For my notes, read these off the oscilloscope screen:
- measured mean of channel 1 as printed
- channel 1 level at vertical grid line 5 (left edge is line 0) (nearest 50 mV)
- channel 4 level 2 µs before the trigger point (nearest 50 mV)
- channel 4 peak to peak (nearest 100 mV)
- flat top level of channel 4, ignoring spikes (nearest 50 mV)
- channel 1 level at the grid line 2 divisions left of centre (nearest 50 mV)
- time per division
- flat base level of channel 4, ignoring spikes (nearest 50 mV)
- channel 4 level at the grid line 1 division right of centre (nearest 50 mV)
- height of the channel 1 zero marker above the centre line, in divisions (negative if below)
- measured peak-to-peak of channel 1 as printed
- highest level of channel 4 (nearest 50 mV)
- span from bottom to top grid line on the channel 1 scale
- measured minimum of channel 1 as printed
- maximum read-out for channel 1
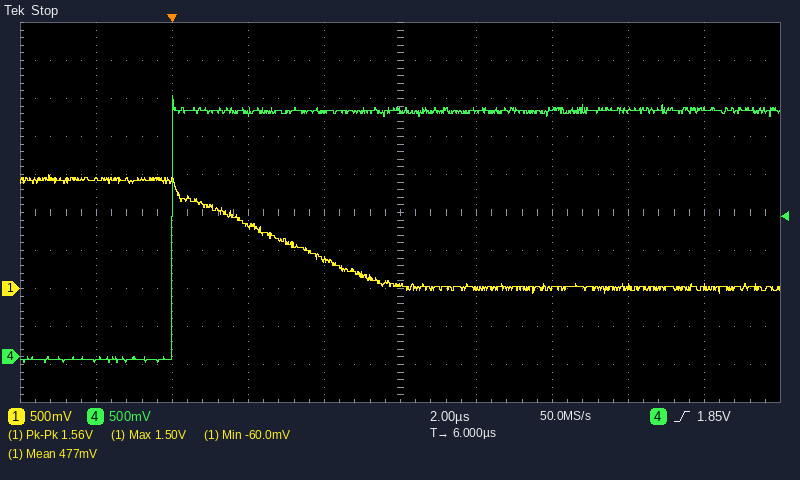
477 mV
50 mV
-50 mV
3.50 V
3.25 V
800 mV
2 µs
-50 mV
3.25 V
-2.0 div
1.56 V
3.45 V
5 V
-60.0 mV
1.50 V
